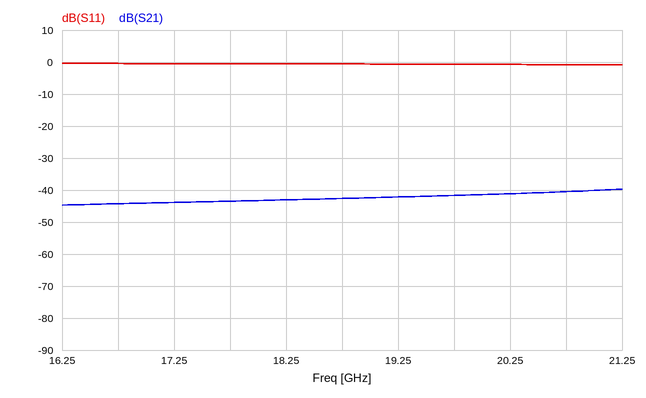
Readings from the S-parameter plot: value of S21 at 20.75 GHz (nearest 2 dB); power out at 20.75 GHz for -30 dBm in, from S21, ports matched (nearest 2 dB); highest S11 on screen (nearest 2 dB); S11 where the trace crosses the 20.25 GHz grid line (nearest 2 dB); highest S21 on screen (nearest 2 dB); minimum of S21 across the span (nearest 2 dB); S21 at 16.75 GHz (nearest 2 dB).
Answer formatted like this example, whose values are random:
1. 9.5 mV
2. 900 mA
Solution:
1. -40 dB
2. -70 dBm
3. 0 dB
4. 0 dB
5. -40 dB
6. -44 dB
7. -44 dB
